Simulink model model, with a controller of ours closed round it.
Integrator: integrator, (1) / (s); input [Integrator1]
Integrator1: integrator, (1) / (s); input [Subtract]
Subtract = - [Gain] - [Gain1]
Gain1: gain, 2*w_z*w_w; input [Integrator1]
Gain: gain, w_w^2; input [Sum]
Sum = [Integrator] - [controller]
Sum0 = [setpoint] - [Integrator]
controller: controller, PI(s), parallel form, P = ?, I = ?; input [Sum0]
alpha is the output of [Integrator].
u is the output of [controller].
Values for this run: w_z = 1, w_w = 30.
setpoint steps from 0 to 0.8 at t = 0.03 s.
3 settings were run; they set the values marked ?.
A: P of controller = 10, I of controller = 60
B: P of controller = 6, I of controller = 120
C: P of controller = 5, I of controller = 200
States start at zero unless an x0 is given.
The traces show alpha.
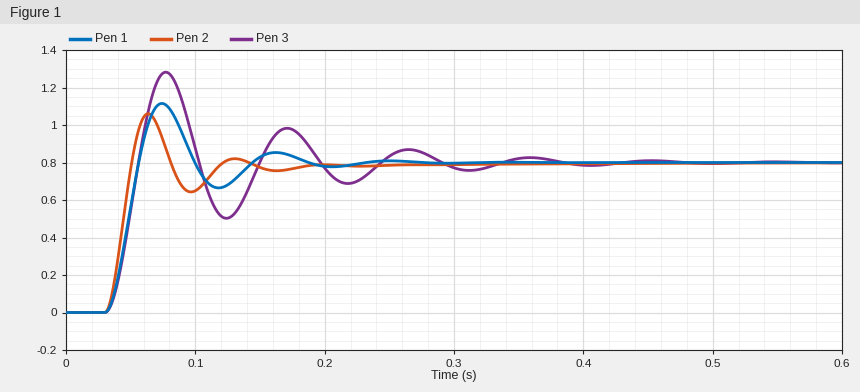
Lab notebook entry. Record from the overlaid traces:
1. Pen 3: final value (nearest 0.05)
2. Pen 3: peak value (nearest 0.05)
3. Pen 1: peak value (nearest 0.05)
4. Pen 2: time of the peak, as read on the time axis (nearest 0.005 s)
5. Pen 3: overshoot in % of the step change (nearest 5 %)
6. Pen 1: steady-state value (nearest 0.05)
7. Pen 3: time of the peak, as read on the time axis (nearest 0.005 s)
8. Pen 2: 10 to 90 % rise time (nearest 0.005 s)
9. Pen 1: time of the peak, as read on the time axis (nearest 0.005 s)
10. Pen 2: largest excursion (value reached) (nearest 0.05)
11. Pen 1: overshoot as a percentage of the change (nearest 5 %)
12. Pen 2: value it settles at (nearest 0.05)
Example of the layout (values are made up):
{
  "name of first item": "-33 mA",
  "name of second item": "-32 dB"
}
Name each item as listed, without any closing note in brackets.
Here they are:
{
  "Pen 3: final value": "0.80",
  "Pen 3: peak value": "1.30",
  "Pen 1: peak value": "1.10",
  "Pen 2: time of the peak, as read on the time axis": "0.065 s",
  "Pen 3: overshoot in % of the step change": "60 %",
  "Pen 1: steady-state value": "0.80",
  "Pen 3: time of the peak, as read on the time axis": "0.075 s",
  "Pen 2: 10 to 90 % rise time": "0.015 s",
  "Pen 1: time of the peak, as read on the time axis": "0.075 s",
  "Pen 2: largest excursion (value reached)": "1.05",
  "Pen 1: overshoot as a percentage of the change": "40 %",
  "Pen 2: value it settles at": "0.80"
}
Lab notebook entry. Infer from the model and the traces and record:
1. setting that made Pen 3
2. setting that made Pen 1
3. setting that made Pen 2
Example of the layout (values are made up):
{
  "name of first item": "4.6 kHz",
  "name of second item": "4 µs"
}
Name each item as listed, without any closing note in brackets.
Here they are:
{
  "setting that made Pen 3": "C",
  "setting that made Pen 1": "B",
  "setting that made Pen 2": "A"
}
